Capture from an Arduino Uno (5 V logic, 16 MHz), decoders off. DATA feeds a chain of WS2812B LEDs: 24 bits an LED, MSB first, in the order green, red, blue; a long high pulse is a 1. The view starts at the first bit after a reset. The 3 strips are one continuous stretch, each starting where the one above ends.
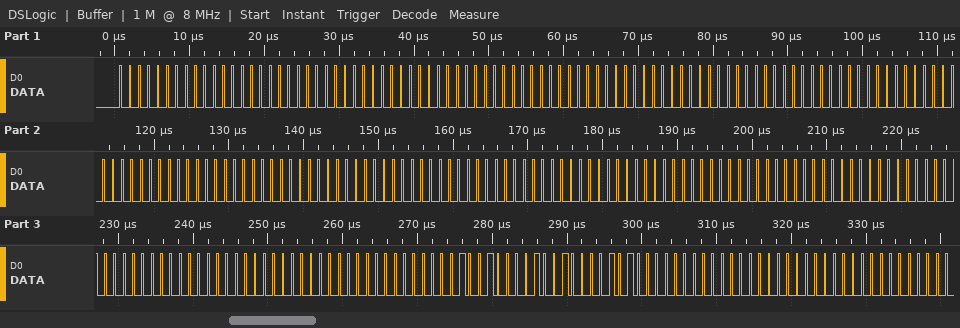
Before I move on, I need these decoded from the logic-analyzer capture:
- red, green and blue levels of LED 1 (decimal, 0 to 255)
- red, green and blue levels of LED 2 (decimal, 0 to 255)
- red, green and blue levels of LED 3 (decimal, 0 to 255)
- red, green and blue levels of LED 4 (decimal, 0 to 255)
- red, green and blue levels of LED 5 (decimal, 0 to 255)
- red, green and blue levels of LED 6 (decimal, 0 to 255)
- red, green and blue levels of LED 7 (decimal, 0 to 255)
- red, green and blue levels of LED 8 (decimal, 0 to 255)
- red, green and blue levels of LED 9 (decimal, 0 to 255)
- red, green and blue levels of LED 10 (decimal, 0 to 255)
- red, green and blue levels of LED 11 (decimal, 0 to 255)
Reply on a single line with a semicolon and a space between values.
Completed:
0, 0, 0; 0, 0, 0; 0, 0, 0; 0, 0, 0; 0, 0, 0; 0, 0, 0; 0, 0, 0; 0, 0, 0; 0, 0, 0; 9, 9, 10; 0, 0, 0
